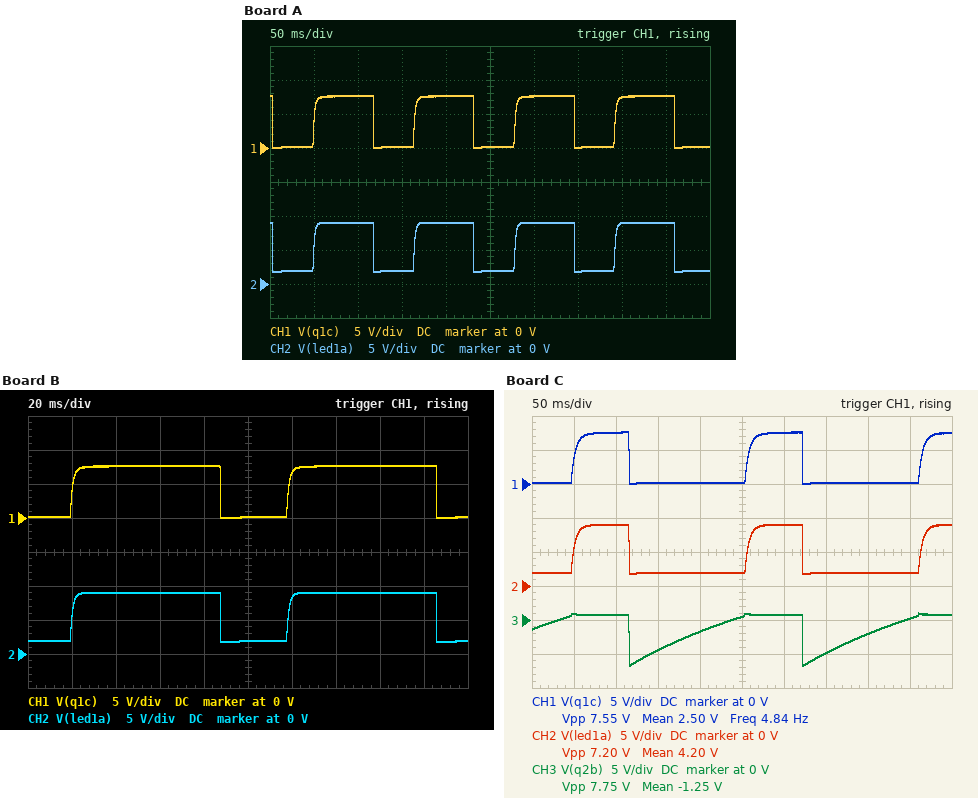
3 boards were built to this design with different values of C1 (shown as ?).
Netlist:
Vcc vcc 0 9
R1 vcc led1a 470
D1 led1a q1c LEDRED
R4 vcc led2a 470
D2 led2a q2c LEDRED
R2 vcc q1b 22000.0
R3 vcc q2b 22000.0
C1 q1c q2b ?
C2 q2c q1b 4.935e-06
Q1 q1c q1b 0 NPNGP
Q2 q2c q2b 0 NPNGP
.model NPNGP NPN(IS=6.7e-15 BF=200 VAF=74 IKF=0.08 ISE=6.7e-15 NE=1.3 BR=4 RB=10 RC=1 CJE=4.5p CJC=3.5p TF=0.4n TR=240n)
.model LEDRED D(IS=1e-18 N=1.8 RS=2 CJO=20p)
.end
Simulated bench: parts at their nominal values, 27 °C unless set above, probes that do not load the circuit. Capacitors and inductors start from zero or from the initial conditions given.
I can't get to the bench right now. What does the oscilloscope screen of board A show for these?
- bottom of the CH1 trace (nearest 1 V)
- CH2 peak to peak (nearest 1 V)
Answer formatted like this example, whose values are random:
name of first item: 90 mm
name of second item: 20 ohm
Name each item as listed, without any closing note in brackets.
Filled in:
bottom of the CH1 trace: 0 V
CH2 peak to peak: 7 V
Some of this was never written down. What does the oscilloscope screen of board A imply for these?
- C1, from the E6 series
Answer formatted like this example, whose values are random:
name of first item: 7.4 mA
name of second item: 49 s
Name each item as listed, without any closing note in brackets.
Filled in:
C1, from the E6 series: 3.3 µF
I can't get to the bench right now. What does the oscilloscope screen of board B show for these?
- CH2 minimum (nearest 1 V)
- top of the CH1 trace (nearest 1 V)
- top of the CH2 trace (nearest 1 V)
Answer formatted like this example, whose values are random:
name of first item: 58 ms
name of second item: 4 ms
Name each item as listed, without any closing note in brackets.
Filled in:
CH2 minimum: 2 V
top of the CH1 trace: 8 V
top of the CH2 trace: 9 V
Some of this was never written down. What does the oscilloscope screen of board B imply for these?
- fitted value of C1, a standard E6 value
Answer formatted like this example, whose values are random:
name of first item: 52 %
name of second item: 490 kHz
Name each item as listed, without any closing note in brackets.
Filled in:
fitted value of C1, a standard E6 value: 2.2 µF
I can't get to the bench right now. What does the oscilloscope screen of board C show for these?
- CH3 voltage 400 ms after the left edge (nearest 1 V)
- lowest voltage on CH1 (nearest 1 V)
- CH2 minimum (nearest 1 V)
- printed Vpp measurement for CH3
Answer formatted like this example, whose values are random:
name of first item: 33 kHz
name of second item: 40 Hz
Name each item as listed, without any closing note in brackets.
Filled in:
CH3 voltage 400 ms after the left edge: -2 V
lowest voltage on CH1: 0 V
CH2 minimum: 2 V
printed Vpp measurement for CH3: 7.75 V
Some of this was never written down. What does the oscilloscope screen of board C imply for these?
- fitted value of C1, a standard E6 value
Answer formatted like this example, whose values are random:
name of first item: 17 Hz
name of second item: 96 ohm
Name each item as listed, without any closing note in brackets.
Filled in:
fitted value of C1, a standard E6 value: 10 µF
